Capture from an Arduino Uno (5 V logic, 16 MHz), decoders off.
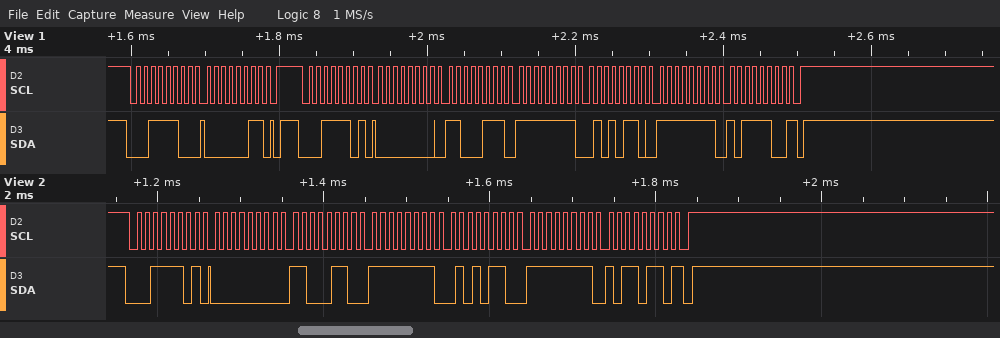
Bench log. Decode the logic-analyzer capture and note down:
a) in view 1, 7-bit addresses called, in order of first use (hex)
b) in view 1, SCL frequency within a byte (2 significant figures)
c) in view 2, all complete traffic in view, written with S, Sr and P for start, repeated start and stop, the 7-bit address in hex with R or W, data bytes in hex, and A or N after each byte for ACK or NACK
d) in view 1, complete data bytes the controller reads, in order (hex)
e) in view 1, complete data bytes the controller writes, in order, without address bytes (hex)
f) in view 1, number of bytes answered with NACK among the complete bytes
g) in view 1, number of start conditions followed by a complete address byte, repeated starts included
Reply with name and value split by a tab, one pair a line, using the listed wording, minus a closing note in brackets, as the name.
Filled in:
in view 1, 7-bit addresses called, in order of first use	0x1E
in view 1, SCL frequency within a byte	100 kHz
in view 2, all complete traffic in view, written with S, Sr and P for start, repeated start and stop, the 7-bit address in hex with R or W, data bytes in hex, and A or N after each byte for ACK or NACK	S 1ER A 00 A C6 A FF A 56 A FF A B6 N P
in view 1, complete data bytes the controller reads, in order	00 C7 FF 56 FF BC
in view 1, complete data bytes the controller writes, in order, without address bytes	03
in view 1, number of bytes answered with NACK among the complete bytes	1
in view 1, number of start conditions followed by a complete address byte, repeated starts included	2
